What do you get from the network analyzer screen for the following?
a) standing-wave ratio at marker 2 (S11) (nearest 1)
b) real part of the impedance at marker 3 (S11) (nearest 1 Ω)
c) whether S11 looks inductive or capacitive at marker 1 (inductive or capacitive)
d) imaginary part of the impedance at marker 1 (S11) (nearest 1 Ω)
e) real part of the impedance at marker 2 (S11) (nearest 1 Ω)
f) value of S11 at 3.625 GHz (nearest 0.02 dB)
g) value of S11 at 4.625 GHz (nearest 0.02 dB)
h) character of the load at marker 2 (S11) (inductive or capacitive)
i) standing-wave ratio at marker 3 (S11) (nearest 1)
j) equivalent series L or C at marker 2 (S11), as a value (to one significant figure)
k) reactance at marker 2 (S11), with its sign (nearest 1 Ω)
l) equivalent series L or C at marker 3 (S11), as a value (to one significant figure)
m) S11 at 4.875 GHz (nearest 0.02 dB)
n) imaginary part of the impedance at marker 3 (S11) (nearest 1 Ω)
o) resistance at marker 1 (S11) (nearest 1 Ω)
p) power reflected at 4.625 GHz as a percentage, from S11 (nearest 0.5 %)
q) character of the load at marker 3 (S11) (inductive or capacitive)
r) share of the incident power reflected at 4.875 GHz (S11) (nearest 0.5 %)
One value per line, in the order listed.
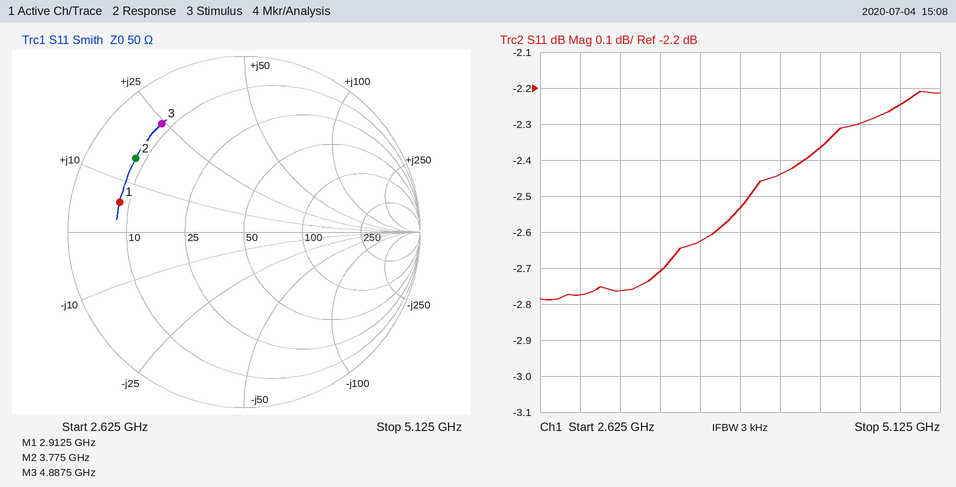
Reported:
7
8 Ω
inductive
+6 Ω
8 Ω
-2.62 dB
-2.30 dB
inductive
8
600 pH
+15 Ω
800 pH
-2.24 dB
+24 Ω
8 Ω
59.0 %
inductive
59.5 %
